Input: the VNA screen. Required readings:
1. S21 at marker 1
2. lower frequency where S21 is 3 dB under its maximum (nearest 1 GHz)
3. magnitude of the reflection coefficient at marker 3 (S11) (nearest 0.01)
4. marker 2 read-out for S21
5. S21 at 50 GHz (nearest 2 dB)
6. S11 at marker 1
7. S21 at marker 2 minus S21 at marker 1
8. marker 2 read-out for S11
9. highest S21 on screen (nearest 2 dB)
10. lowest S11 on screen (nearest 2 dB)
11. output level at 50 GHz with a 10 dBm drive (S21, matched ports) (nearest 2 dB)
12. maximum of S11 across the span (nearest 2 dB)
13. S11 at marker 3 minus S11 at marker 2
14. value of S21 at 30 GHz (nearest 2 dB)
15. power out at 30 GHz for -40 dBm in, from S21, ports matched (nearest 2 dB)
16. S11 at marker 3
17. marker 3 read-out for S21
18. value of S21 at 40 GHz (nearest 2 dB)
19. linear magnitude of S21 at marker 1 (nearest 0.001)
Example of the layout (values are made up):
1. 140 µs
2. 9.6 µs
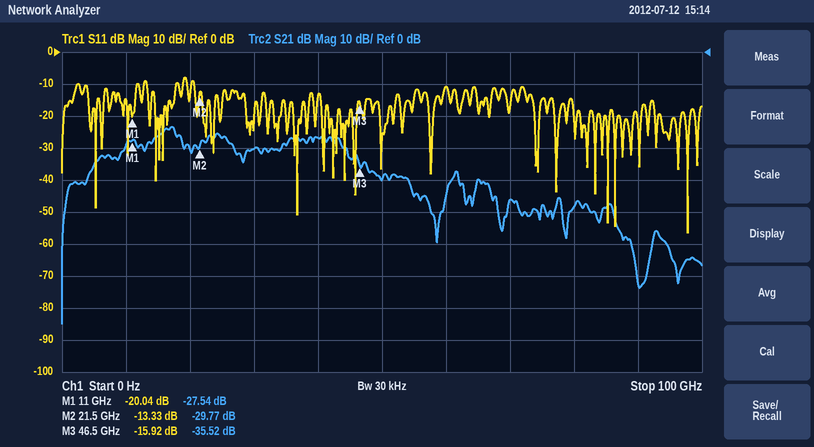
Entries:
1. -27.54 dB
2. 15 GHz
3. 0.16
4. -29.77 dB
5. -40 dB
6. -20.04 dB
7. -2.23 dB
8. -13.33 dB
9. -24 dB
10. -56 dB
11. -30 dBm
12. -8 dB
13. -2.59 dB
14. -30 dB
15. -70 dBm
16. -15.92 dB
17. -35.52 dB
18. -26 dB
19. 0.042
